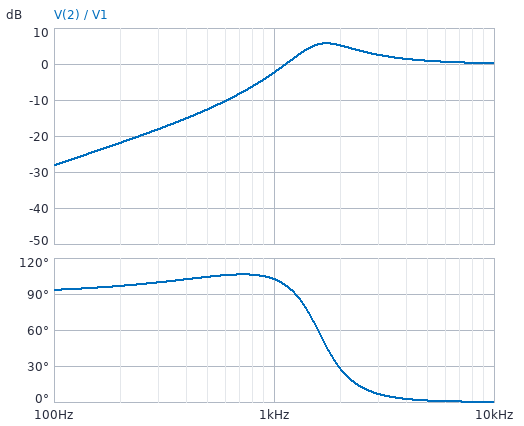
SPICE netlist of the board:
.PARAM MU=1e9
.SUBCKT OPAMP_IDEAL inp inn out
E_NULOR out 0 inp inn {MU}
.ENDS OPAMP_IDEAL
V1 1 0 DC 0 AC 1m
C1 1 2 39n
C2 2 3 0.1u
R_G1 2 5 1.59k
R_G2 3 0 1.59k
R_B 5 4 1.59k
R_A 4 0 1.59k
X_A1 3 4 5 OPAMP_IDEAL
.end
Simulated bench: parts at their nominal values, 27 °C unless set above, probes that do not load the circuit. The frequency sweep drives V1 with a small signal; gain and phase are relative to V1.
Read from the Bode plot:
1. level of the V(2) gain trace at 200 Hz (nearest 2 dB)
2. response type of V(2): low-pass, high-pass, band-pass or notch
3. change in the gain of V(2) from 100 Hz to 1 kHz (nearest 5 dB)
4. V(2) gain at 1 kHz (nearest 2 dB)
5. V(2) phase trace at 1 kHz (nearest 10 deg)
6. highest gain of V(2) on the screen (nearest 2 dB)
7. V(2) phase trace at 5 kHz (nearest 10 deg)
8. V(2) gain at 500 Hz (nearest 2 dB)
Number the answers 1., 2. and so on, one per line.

1. -22 dB
2. high-pass
3. 25 dB
4. -2 dB
5. 100 deg
6. 6 dB
7. 0 deg
8. -12 dB
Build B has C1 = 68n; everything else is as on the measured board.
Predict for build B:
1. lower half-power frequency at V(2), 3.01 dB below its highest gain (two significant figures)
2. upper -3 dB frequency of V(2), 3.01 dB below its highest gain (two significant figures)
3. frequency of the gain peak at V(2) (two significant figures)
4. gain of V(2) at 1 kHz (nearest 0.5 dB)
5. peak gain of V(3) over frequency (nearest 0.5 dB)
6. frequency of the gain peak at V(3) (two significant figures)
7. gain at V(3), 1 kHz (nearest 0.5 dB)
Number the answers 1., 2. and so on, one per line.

1. 930 Hz
2. 3.2 kHz
3. 1.4 kHz
4. 2.0 dB
5. 2.5 dB
6. 1.5 kHz
7. -1.0 dB
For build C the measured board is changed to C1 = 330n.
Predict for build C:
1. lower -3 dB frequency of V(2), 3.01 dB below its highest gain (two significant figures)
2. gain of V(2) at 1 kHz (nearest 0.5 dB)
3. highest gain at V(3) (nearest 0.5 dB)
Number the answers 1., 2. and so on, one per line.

1. 290 Hz
2. 1.5 dB
3. 0 dB
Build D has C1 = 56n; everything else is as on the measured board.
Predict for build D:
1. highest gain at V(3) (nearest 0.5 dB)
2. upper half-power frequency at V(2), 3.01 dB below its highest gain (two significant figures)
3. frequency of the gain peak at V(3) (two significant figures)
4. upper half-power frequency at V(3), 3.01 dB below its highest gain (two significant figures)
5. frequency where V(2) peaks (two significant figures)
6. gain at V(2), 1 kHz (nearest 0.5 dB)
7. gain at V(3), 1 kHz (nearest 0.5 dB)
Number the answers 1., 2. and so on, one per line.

1. 3.0 dB
2. 3.0 kHz
3. 1.6 kHz
4. 8.3 kHz
5. 1.5 kHz
6. 1.0 dB
7. -2.0 dB
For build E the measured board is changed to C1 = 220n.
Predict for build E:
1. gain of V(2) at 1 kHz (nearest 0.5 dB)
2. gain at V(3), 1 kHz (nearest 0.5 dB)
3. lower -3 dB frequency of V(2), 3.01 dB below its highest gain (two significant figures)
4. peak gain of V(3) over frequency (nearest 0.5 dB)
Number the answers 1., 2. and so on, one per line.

1. 2.0 dB
2. -1.0 dB
3. 410 Hz
4. 0 dB
